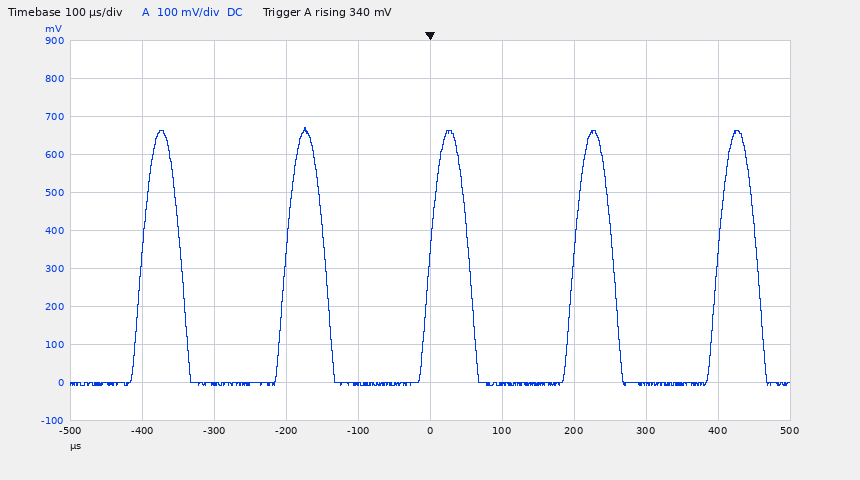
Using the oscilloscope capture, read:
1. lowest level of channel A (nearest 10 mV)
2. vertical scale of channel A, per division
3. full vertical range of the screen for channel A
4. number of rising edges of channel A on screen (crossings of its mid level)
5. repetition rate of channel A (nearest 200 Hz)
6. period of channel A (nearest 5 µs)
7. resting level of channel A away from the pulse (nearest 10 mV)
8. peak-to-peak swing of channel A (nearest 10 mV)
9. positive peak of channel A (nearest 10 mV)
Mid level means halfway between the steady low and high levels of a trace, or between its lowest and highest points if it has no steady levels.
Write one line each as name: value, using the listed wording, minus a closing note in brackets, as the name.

lowest level of channel A: -10 mV
vertical scale of channel A, per division: 100 mV
full vertical range of the screen for channel A: 1 V
number of rising edges of channel A on screen: 5
repetition rate of channel A: 5.0 kHz
period of channel A: 200 µs
resting level of channel A away from the pulse: 0 mV
peak-to-peak swing of channel A: 680 mV
positive peak of channel A: 670 mV
